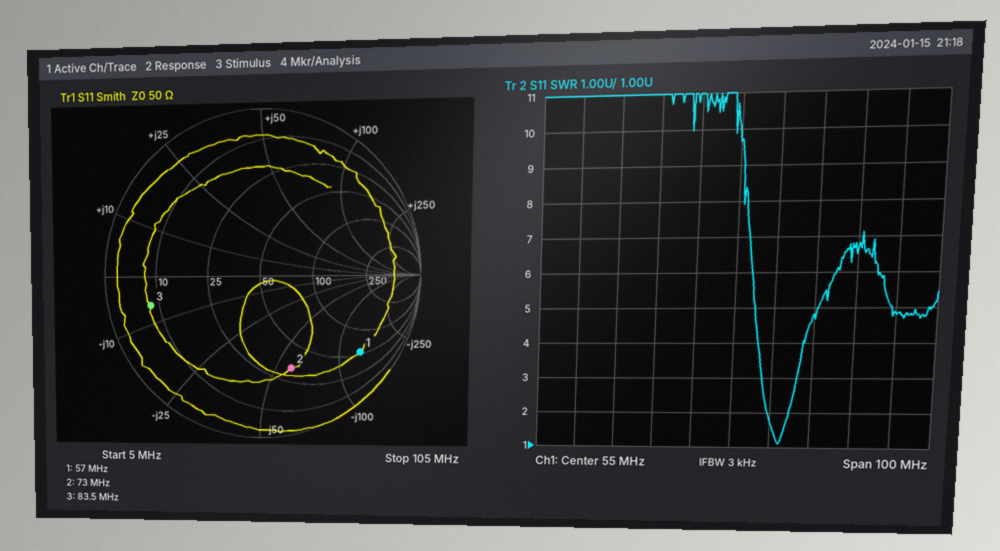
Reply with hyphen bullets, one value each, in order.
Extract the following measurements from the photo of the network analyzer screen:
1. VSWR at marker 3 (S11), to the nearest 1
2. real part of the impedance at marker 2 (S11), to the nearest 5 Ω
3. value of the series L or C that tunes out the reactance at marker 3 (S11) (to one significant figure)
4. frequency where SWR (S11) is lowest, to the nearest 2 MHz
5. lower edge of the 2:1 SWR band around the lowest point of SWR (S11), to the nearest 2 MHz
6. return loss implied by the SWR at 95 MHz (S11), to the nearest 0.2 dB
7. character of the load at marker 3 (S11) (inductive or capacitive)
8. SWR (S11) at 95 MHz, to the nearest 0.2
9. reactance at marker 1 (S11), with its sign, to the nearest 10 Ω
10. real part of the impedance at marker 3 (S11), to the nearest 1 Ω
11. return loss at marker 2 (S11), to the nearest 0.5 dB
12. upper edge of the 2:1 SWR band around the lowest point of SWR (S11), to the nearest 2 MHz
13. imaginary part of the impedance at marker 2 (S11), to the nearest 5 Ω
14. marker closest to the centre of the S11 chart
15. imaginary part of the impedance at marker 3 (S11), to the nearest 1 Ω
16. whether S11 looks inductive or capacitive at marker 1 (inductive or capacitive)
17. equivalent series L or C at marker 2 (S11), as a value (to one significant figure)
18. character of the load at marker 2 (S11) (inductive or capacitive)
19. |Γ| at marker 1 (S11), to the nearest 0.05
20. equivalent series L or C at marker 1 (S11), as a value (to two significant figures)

- 6
- 35 Ω
- 10 nH
- 68 MHz
- 64 MHz
- 3.6 dB
- capacitive
- 4.8
- -130 Ω
- 8 Ω
- 4.5 dB
- 70 MHz
- -60 Ω
- marker 2
- -6 Ω
- capacitive
- 40 pF
- capacitive
- 0.80
- 21 pF
